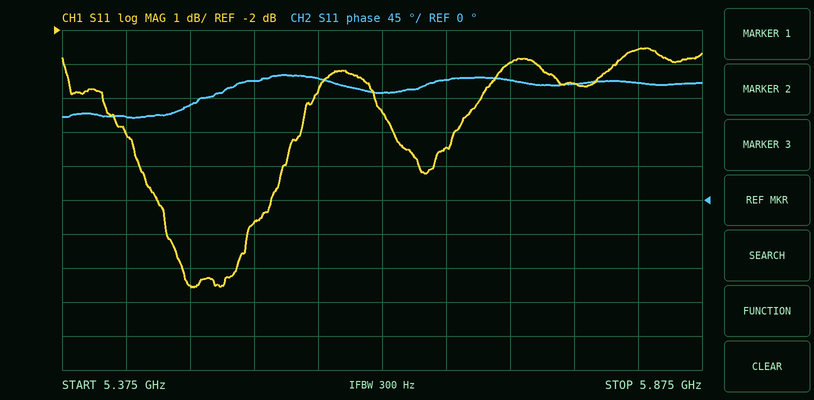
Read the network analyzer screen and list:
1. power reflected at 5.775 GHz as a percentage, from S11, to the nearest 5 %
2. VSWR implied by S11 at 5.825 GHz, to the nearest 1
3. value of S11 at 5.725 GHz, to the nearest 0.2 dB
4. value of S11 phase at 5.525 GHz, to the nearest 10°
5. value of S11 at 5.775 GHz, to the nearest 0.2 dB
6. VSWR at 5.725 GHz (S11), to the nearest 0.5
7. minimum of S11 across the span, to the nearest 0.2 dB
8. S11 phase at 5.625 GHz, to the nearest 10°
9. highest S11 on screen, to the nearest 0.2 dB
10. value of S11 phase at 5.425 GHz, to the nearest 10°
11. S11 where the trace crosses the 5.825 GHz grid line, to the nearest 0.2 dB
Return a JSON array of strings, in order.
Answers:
["45 %", "7", "-3.0 dB", "160°", "-3.6 dB", "6.0", "-9.6 dB", "140°", "-2.6 dB", "110°", "-2.6 dB"]
